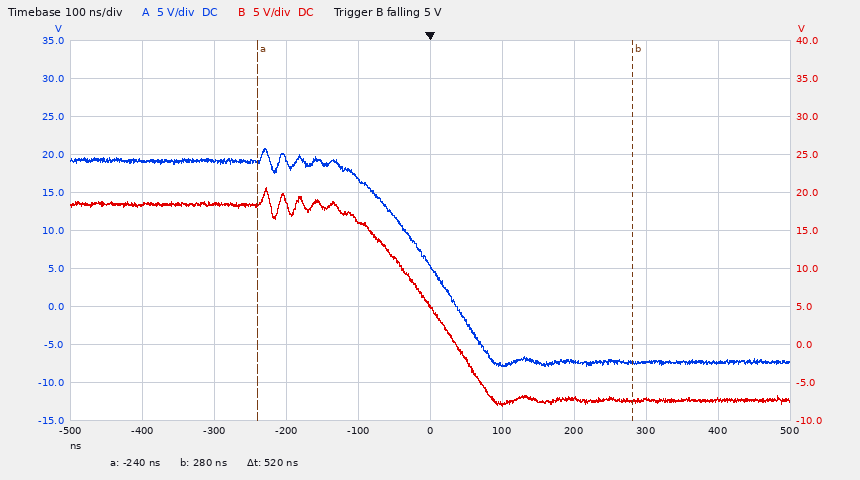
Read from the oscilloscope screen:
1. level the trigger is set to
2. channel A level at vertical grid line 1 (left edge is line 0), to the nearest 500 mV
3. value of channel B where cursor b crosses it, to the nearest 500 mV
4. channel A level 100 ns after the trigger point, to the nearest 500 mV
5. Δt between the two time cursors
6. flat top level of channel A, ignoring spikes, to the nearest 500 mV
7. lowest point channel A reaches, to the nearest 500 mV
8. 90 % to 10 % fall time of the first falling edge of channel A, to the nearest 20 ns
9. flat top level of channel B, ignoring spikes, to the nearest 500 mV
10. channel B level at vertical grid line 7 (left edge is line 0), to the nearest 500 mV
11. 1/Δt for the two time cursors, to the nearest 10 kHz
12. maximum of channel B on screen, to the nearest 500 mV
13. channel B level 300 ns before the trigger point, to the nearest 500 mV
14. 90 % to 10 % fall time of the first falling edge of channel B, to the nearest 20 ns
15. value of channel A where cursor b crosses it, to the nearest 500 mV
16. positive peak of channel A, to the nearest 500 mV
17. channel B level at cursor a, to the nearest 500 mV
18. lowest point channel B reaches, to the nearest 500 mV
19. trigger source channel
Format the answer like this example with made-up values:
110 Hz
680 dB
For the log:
5 V
19.0 V
-7.5 V
-7.5 V
520 ns
19.0 V
-8.0 V
160 ns
18.5 V
-7.0 V
1.92 MHz
20.5 V
18.5 V
160 ns
-7.5 V
21.0 V
18.5 V
-8.0 V
channel B
